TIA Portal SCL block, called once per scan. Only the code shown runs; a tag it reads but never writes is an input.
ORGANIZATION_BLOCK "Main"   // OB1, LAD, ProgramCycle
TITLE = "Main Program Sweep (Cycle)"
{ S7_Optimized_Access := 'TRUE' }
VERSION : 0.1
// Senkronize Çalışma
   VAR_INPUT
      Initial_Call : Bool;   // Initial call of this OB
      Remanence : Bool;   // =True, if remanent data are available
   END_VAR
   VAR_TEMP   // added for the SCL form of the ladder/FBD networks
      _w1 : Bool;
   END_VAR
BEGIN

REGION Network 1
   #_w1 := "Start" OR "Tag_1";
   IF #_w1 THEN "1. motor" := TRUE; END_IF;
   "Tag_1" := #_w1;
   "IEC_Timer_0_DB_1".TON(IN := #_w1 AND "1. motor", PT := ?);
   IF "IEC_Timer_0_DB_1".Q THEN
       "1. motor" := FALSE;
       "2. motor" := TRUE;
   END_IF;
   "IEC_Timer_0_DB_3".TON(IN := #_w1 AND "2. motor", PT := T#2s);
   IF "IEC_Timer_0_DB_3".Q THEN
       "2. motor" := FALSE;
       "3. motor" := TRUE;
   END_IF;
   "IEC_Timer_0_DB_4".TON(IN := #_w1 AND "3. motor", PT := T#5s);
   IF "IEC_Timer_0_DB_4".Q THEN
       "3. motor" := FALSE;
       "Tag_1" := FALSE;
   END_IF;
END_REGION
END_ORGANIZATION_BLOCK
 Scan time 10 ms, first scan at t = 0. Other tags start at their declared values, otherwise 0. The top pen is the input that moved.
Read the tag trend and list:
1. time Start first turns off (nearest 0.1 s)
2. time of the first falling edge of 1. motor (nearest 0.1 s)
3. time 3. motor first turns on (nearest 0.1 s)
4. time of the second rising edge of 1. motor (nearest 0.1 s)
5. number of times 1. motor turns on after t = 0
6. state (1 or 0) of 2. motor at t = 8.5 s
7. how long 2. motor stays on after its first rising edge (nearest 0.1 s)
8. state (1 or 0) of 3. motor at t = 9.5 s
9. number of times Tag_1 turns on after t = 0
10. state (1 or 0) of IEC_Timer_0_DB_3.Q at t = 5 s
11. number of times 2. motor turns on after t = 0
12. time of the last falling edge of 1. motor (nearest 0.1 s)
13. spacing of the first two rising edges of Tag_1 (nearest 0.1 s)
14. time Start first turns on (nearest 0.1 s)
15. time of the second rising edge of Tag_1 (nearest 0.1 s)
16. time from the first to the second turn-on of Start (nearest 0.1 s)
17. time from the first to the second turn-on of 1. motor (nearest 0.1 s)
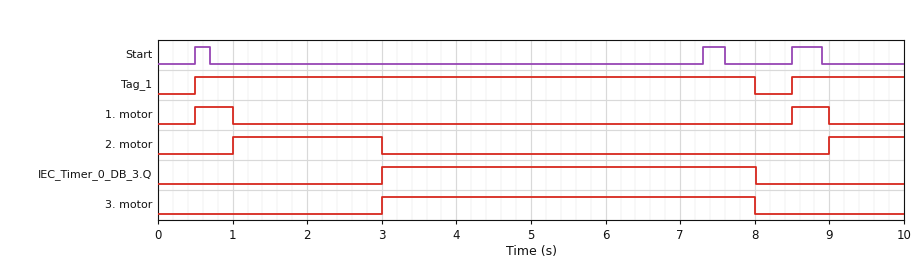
0.7 s
1.0 s
3.0 s
8.5 s
2
0
2.0 s
0
2
1
2
9.0 s
8.0 s
0.5 s
8.5 s
6.8 s
8.0 s
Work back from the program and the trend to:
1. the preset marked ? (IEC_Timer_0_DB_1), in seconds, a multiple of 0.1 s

0.5 s
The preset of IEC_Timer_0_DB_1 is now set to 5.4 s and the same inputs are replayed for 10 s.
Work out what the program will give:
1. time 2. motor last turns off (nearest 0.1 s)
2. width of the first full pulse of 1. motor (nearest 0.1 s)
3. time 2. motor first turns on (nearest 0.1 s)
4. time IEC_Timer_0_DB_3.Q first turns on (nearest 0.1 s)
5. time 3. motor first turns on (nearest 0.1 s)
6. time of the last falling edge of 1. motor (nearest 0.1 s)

7.9 s
5.4 s
5.9 s
7.9 s
7.9 s
5.9 s
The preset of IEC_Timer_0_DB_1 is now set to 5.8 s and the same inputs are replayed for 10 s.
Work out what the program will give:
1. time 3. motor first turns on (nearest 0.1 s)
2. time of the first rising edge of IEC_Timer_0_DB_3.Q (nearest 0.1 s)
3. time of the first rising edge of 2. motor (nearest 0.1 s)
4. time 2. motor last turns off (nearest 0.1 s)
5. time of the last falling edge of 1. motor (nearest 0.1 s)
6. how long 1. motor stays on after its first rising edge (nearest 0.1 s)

8.3 s
8.3 s
6.3 s
8.3 s
6.3 s
5.8 s
